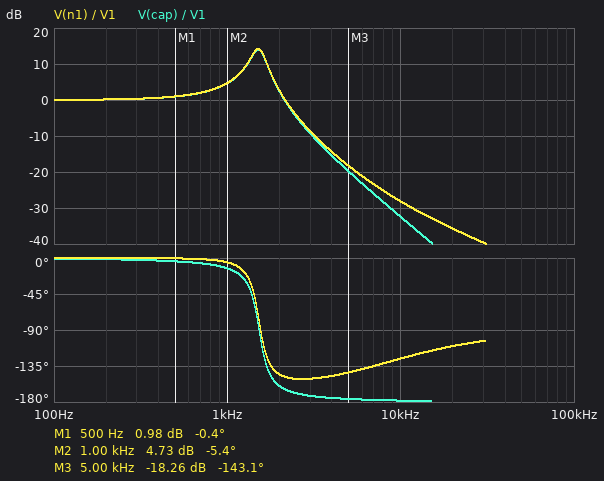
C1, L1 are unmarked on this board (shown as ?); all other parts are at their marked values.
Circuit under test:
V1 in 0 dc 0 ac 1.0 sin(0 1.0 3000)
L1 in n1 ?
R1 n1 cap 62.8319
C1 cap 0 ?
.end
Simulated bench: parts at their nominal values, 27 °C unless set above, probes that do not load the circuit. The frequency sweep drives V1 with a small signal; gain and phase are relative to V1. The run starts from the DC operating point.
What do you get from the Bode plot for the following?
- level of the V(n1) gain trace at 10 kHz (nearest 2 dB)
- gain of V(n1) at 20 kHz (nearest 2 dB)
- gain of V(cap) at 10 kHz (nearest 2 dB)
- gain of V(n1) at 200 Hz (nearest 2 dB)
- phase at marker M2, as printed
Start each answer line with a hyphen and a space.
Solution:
- -28 dB
- -36 dB
- -32 dB
- 0 dB
- -5.4 deg
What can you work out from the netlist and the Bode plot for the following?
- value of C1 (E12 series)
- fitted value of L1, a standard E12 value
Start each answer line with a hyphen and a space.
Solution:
- 330 nF
- 33 mH
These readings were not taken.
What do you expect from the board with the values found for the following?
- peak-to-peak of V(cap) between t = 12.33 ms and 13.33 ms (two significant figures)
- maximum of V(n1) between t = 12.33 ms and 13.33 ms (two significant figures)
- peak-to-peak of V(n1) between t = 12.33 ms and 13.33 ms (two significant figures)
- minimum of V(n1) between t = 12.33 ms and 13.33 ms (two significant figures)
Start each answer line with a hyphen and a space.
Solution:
- 690 mV
- 370 mV
- 740 mV
- -370 mV
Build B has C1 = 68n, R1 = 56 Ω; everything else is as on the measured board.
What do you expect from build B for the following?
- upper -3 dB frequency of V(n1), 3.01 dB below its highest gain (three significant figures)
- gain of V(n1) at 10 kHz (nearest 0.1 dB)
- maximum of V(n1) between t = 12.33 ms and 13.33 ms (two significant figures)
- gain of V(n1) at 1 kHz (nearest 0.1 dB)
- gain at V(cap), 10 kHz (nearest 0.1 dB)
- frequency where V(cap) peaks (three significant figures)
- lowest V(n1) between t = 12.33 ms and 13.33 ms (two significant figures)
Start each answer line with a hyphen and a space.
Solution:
- 3.49 kHz
- -17.7 dB
- 4.7 V
- 0.8 dB
- -17.9 dB
- 3.35 kHz
- -4.7 V
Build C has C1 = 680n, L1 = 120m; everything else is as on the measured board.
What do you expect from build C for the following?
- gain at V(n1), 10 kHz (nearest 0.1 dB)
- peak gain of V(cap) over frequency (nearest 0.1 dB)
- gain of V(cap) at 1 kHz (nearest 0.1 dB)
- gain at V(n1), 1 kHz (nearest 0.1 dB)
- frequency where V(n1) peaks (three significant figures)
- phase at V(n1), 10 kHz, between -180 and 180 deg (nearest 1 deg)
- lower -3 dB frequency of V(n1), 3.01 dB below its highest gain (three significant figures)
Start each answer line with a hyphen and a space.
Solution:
- -41.0 dB
- 16.5 dB
- -7.0 dB
- -6.7 dB
- 554 Hz
- -110 deg
- 511 Hz
